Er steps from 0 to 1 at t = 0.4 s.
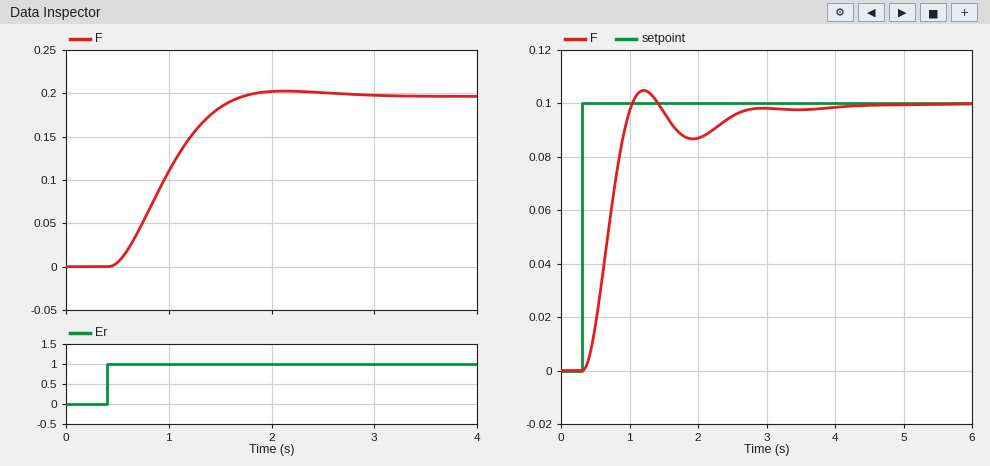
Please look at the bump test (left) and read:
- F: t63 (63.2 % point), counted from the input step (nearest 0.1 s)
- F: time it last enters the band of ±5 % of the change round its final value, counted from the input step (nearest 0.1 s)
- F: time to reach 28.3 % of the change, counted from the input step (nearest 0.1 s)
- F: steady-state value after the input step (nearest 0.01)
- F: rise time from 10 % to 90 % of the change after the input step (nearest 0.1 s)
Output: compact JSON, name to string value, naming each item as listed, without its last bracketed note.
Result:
{"F: t63 (63.2 % point), counted from the input step": "0.7 s", "F: time it last enters the band of ±5 % of the change round its final value, counted from the input step": "1.1 s", "F: time to reach 28.3 % of the change, counted from the input step": "0.4 s", "F: steady-state value after the input step": "0.20", "F: rise time from 10 % to 90 % of the change after the input step": "0.8 s"}
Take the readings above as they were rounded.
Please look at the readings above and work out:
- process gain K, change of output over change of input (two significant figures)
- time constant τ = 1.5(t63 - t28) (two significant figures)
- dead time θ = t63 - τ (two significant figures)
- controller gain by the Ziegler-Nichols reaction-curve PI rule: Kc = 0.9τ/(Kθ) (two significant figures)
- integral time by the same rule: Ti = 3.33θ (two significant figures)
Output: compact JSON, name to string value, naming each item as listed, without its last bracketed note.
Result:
{"process gain K, change of output over change of input": "0.20", "time constant τ = 1.5(t63 - t28)": "0.45 s", "dead time θ = t63 - τ": "0.25 s", "controller gain by the Ziegler-Nichols reaction-curve PI rule: Kc = 0.9τ/(Kθ)": "8.1", "integral time by the same rule: Ti = 3.33θ": "0.83 s"}
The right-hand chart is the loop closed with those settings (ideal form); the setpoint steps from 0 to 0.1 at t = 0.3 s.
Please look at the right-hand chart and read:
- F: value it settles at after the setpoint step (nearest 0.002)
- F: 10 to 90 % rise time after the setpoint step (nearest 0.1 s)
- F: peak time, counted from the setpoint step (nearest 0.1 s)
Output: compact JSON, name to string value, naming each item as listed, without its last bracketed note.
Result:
{"F: value it settles at after the setpoint step": "0.100", "F: 10 to 90 % rise time after the setpoint step": "0.5 s", "F: peak time, counted from the setpoint step": "0.9 s"}
